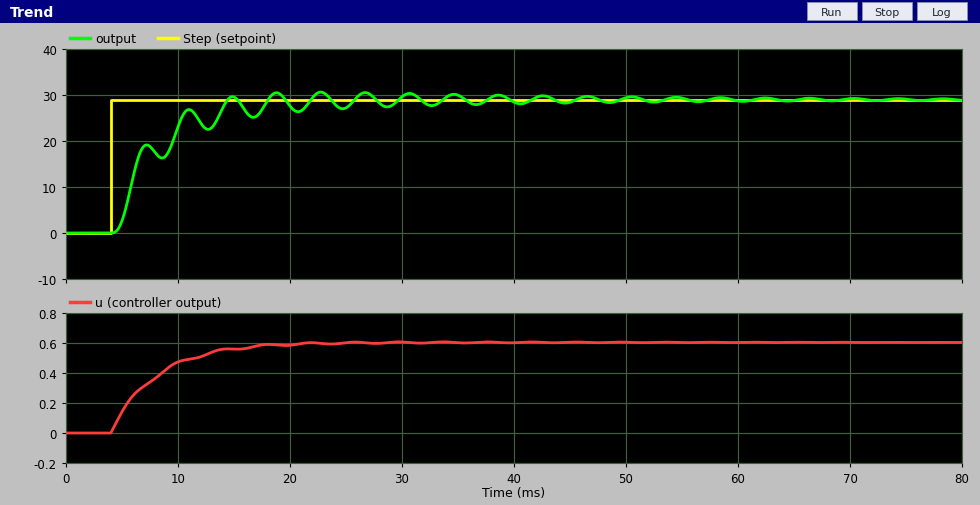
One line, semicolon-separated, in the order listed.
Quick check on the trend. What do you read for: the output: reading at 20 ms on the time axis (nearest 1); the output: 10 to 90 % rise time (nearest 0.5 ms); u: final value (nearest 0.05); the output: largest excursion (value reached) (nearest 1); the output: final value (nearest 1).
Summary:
28; 5.5 ms; 0.60; 31; 29
